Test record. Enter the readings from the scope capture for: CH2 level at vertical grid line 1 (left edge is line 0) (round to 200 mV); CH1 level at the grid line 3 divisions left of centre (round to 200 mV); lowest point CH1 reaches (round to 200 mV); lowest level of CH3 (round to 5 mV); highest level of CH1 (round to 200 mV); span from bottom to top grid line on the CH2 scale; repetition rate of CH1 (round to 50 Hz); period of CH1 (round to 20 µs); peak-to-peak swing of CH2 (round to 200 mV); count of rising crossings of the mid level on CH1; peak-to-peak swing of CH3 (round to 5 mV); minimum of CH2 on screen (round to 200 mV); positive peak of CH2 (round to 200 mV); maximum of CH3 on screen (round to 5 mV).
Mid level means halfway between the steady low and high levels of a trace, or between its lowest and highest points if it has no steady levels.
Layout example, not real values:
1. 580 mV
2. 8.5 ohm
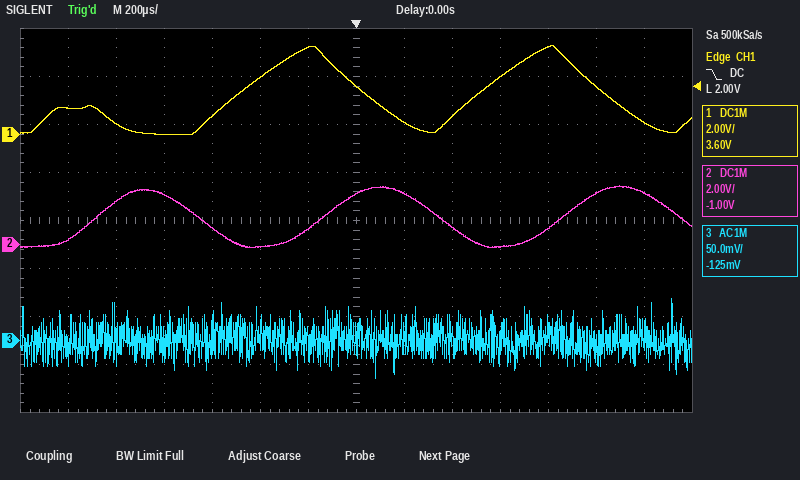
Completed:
1. 200 mV
2. 800 mV
3. 0.0 V
4. -40 mV
5. 3.6 V
6. 16 V
7. 1.00 kHz
8. 1.00 ms
9. 2.6 V
10. 2
11. 85 mV
12. -200 mV
13. 2.4 V
14. 45 mV
